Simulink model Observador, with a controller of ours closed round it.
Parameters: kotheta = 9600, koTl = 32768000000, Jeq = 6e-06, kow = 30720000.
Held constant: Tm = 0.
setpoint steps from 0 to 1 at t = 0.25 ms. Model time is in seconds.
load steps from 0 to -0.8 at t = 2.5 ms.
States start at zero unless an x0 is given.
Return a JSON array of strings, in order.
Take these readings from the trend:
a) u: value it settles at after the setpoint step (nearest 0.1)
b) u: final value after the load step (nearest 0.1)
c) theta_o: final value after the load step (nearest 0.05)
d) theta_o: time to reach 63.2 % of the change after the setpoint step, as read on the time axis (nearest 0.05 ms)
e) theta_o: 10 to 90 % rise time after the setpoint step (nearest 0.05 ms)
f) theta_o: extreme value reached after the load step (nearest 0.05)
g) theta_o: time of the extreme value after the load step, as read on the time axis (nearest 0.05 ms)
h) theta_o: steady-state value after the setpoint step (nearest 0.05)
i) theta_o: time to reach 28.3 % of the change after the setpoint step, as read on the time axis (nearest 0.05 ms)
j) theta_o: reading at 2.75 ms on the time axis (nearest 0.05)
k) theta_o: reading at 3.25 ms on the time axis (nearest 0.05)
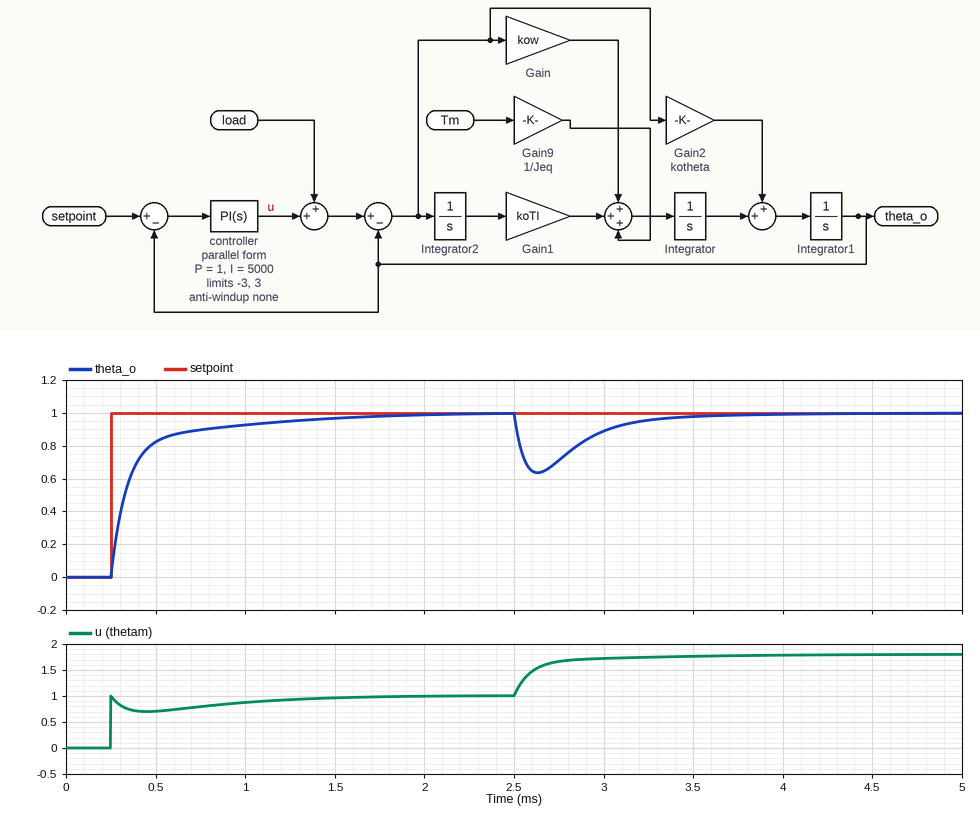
["1.0", "1.8", "1.00", "0.35 ms", "0.50 ms", "0.65", "2.65 ms", "1.00", "0.30 ms", "0.70", "0.95"]
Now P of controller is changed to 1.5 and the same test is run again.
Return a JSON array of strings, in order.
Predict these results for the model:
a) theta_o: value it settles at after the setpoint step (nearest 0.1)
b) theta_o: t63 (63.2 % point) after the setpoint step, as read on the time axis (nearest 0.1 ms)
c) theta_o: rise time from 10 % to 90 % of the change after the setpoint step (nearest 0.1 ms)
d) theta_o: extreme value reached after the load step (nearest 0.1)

["1.0", "0.3 ms", "0.6 ms", "0.7"]
